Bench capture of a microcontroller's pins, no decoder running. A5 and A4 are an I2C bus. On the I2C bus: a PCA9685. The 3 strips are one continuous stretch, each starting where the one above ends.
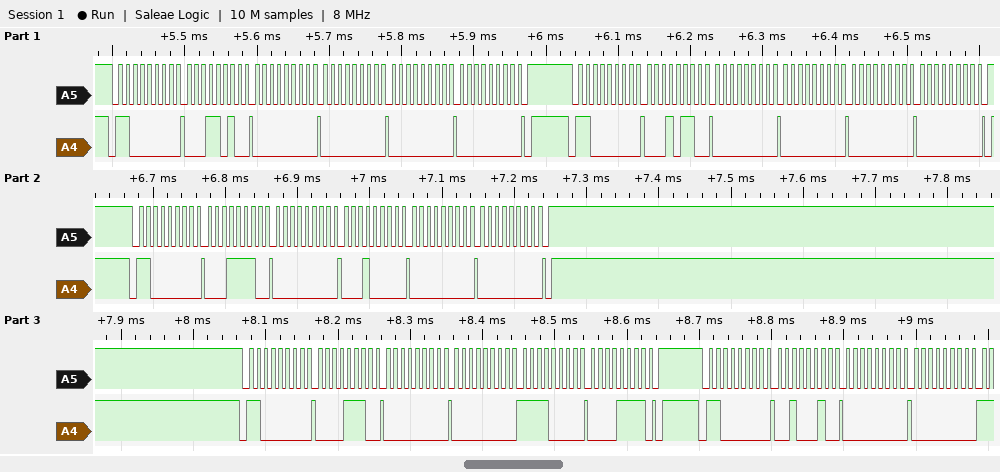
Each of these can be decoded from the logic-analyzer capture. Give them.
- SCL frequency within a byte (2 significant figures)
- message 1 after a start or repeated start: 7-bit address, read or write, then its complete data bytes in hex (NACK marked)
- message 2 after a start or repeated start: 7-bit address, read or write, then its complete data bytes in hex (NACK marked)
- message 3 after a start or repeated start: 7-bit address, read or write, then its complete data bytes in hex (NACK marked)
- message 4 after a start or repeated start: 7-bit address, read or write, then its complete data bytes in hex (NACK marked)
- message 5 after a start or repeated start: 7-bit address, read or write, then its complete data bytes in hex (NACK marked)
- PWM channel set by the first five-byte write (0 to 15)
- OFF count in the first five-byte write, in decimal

100 kHz
0x60 write: 1A 00 00 00 00
0x60 write: 16 00 00 00 00
0x60 write: 1E 00 10 00 00
0x60 write: 0E 00 00 F0 0F
0x60 write: 22 00 00
5
0
